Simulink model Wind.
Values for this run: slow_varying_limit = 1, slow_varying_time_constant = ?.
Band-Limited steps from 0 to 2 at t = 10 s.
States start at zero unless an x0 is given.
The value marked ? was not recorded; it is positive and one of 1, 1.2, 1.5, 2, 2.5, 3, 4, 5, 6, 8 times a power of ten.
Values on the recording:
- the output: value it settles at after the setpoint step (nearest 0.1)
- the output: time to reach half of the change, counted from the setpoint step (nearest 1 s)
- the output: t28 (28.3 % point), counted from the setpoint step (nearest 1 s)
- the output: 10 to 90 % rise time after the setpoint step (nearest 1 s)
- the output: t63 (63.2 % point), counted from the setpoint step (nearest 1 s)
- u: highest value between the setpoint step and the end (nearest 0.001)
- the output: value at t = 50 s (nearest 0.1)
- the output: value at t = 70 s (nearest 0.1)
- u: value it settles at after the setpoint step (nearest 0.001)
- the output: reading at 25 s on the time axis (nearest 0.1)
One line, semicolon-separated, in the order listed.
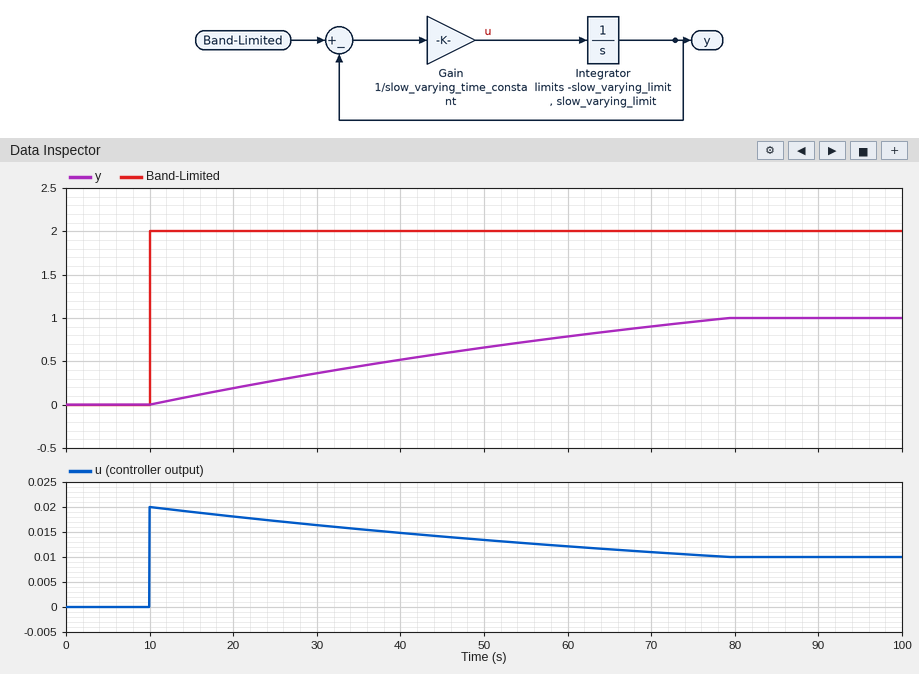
1.0; 29 s; 15 s; 55 s; 38 s; 0.020; 0.7; 0.9; 0.010; 0.3
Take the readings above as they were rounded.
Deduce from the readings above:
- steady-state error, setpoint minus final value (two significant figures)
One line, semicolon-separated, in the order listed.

1.0
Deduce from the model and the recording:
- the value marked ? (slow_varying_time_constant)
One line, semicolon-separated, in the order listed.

100
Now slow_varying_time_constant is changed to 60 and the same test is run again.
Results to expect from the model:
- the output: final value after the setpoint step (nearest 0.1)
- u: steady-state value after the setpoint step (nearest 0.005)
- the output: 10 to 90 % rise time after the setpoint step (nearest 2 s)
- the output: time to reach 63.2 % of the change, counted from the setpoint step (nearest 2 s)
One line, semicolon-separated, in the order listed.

1.0; 0.015; 32 s; 22 s
